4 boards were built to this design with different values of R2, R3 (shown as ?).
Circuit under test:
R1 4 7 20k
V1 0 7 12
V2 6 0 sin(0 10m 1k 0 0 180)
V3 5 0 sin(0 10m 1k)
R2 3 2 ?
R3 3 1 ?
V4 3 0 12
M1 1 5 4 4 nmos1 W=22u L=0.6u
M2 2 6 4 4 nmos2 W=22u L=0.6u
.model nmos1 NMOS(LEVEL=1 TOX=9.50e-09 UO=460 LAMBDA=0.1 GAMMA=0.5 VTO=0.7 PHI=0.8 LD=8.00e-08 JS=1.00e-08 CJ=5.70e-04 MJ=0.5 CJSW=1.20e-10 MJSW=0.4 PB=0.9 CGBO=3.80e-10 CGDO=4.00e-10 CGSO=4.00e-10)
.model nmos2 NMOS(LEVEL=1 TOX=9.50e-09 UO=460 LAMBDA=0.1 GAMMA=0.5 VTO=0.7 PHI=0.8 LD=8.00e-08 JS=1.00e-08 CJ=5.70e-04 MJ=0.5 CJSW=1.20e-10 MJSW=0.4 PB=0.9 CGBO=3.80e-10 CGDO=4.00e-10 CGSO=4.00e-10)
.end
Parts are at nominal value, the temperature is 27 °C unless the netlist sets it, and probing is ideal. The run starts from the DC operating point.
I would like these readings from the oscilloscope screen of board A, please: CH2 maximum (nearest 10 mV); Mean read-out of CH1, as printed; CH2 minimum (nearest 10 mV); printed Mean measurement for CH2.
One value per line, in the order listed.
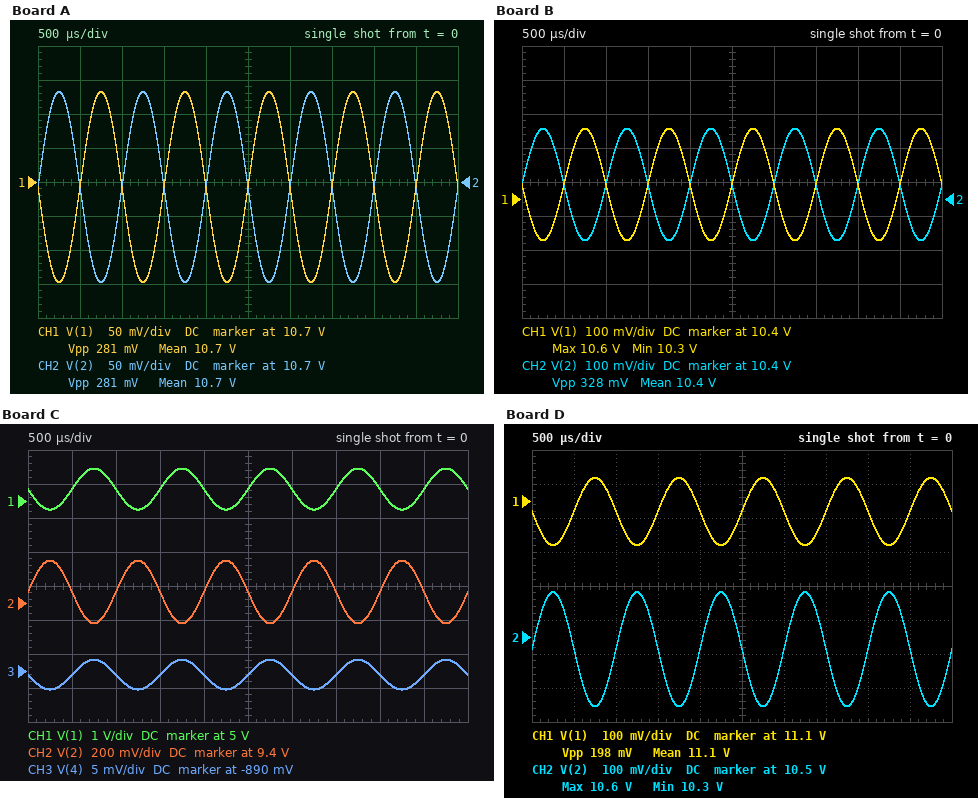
10.83 V
10.7 V
10.55 V
10.7 V
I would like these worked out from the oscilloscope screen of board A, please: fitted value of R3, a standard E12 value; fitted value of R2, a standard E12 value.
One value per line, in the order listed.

4.7 kΩ
4.7 kΩ
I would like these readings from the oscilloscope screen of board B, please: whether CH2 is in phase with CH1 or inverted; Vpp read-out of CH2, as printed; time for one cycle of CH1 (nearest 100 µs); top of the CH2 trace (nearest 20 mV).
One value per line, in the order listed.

inverted
328 mV
1.0 ms
10.60 V
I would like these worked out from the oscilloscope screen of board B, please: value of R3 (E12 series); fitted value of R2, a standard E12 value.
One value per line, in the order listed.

5.6 kΩ
5.6 kΩ
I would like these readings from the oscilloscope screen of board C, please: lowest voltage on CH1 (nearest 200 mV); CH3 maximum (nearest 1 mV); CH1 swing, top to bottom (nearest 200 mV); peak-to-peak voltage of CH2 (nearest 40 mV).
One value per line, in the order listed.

4.8 V
-888 mV
1.2 V
360 mV
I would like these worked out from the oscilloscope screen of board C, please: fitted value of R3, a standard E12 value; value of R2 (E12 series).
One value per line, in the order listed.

27 kΩ
8.2 kΩ
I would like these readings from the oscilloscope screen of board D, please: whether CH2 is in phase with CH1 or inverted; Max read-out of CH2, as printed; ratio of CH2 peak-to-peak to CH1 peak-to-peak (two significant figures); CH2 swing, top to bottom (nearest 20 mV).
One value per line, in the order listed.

inverted
10.6 V
1.7
340 mV
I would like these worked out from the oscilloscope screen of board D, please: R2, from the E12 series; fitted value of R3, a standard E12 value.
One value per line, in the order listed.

5.6 kΩ
3.3 kΩ
